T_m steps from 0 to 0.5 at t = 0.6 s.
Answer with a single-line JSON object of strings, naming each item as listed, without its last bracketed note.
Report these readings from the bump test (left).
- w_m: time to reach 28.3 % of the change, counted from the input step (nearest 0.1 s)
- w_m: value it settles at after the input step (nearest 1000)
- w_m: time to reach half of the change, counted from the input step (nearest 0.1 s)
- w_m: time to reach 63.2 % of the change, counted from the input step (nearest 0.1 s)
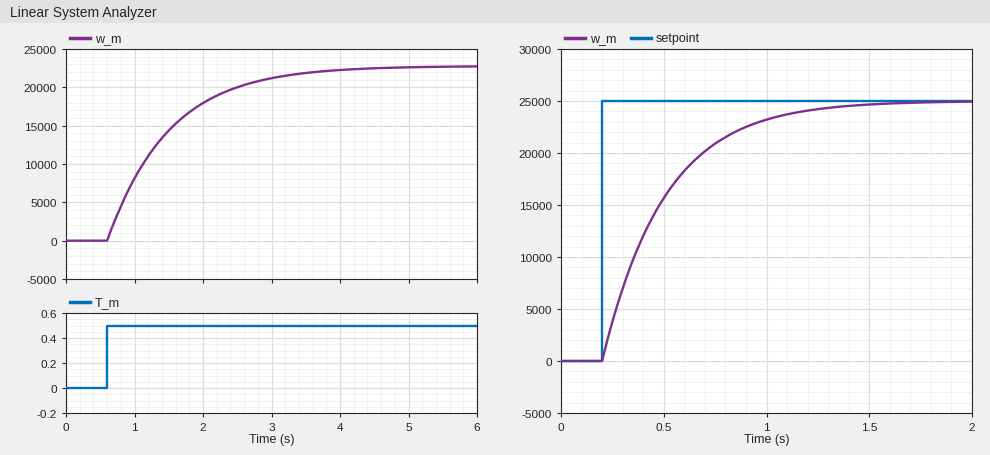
{"w_m: time to reach 28.3 % of the change, counted from the input step": "0.3 s", "w_m: value it settles at after the input step": "23000", "w_m: time to reach half of the change, counted from the input step": "0.6 s", "w_m: time to reach 63.2 % of the change, counted from the input step": "0.9 s"}
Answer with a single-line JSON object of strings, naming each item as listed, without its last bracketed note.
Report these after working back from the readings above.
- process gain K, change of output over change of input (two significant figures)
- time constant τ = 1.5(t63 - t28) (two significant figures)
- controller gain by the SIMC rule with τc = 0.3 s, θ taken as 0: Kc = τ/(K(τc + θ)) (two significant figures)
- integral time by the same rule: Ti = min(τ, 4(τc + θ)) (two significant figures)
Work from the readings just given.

{"process gain K, change of output over change of input": "46000", "time constant τ = 1.5(t63 - t28)": "0.90 s", "controller gain by the SIMC rule with τc = 0.3 s, θ taken as 0: Kc = τ/(K(τc + θ))": "0.000065", "integral time by the same rule: Ti = min(τ, 4(τc + θ))": "0.90 s"}
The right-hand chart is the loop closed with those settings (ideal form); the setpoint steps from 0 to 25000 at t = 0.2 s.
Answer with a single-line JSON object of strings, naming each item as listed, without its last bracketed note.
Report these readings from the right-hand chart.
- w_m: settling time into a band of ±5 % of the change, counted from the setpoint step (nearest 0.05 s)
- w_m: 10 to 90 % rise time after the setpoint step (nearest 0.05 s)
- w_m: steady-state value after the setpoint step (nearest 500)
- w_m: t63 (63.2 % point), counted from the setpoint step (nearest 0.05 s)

{"w_m: settling time into a band of ±5 % of the change, counted from the setpoint step": "0.90 s", "w_m: 10 to 90 % rise time after the setpoint step": "0.65 s", "w_m: steady-state value after the setpoint step": "25000", "w_m: t63 (63.2 % point), counted from the setpoint step": "0.30 s"}
